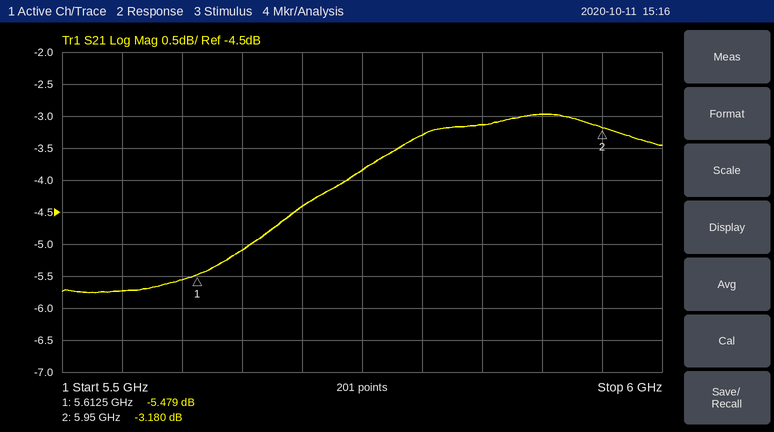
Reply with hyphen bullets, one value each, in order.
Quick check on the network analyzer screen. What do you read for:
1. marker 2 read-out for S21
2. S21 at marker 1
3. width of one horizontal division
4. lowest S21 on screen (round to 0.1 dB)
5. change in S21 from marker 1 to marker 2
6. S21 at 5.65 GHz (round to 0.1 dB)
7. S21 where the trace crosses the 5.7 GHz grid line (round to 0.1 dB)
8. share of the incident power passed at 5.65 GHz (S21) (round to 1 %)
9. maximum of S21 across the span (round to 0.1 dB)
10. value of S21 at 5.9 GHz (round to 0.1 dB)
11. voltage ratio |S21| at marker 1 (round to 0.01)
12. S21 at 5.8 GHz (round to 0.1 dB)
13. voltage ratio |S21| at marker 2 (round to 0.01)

- -3.180 dB
- -5.479 dB
- 50 MHz
- -5.8 dB
- 2.299 dB
- -5.1 dB
- -4.4 dB
- 31 %
- -3.0 dB
- -3.0 dB
- 0.53
- -3.3 dB
- 0.69
